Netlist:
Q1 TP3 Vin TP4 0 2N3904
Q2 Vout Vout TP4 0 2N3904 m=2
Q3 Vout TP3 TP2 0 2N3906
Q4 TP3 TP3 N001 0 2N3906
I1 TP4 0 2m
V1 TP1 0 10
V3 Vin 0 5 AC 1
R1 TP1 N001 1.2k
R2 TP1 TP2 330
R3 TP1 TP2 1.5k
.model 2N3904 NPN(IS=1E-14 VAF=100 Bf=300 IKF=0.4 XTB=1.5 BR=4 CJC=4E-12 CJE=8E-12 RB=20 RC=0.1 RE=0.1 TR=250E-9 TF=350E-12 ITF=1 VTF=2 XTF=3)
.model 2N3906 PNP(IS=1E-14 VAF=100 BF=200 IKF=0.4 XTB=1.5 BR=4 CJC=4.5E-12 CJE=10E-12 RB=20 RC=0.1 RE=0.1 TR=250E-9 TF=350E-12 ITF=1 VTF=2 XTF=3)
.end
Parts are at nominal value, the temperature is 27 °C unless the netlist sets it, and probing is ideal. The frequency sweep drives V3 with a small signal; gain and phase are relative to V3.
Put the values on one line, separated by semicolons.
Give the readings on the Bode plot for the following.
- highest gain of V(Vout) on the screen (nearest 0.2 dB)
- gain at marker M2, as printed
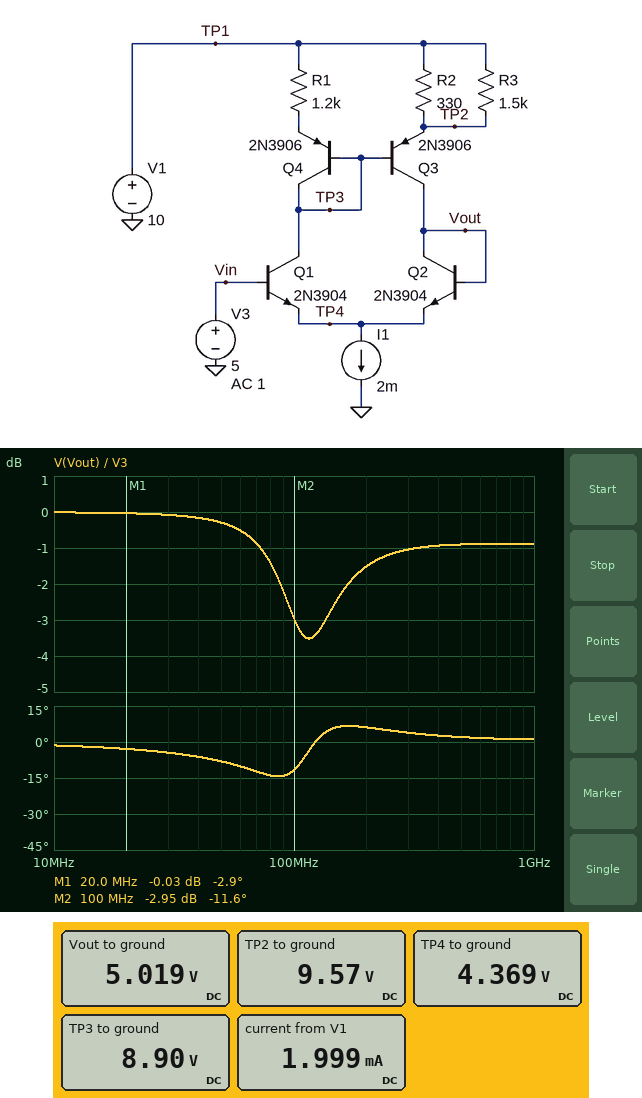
0 dB; -2.95 dB
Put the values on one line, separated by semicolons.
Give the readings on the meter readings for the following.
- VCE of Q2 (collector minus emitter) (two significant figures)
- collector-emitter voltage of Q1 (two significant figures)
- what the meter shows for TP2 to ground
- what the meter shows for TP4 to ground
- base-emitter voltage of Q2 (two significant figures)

650 mV; 4.5 V; 9.57 V; 4.369 V; 650 mV
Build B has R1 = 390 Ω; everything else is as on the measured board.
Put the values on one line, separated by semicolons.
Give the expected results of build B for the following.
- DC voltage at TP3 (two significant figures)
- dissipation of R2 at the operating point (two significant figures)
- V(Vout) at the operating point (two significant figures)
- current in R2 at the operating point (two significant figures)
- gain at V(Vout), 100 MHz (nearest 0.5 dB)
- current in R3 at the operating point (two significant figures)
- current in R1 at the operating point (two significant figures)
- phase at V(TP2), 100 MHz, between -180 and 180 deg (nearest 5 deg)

9.0 V; 300 µW; 5.0 V; 960 µA; -1.0 dB; 210 µA; 830 µA; 90 deg
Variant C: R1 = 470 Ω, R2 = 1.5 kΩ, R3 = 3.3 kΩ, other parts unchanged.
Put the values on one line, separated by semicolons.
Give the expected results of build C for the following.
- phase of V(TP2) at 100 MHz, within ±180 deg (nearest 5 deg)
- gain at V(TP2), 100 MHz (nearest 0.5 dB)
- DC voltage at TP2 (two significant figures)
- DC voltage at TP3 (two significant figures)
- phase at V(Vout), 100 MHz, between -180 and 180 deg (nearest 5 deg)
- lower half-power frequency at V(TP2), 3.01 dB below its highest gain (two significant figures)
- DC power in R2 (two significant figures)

70 deg; -4.0 dB; 9.3 V; 8.7 V; -5 deg; 110 MHz; 290 µW
